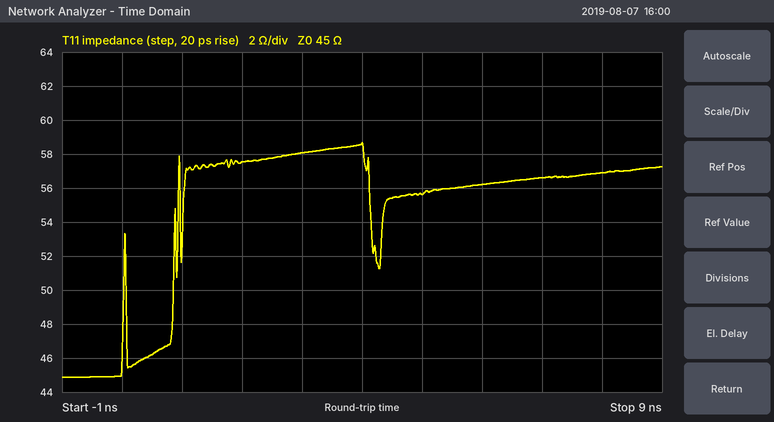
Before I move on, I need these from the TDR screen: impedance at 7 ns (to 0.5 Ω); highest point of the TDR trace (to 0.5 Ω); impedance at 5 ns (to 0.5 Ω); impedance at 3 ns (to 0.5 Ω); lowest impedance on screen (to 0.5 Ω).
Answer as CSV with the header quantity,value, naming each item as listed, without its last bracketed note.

quantity,value
impedance at 7 ns,56.5 Ω
highest point of the TDR trace,58.5 Ω
impedance at 5 ns,55.5 Ω
impedance at 3 ns,58.0 Ω
lowest impedance on screen,45.0 Ω
